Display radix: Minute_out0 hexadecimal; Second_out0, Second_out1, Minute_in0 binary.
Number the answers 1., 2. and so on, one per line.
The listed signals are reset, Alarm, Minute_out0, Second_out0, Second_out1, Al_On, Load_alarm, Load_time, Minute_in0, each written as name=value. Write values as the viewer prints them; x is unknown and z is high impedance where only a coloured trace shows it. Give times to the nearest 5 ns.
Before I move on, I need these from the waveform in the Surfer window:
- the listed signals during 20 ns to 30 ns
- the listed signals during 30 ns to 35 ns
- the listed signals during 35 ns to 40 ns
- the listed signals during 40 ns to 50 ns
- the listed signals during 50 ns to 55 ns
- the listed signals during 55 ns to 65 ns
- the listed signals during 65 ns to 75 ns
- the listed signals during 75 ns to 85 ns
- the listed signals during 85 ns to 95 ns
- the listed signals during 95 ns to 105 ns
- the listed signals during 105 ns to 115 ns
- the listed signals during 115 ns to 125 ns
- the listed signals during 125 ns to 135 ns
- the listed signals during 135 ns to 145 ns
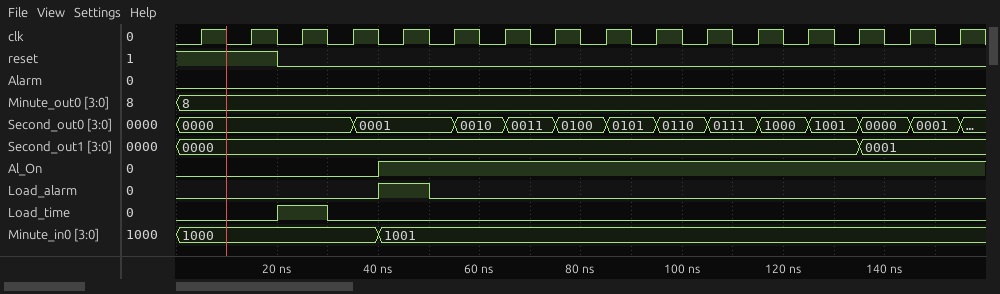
1. reset=0, Alarm=0, Minute_out0=8, Second_out0=0000, Second_out1=0000, Al_On=0, Load_alarm=0, Load_time=1, Minute_in0=1000
2. reset=0, Alarm=0, Minute_out0=8, Second_out0=0000, Second_out1=0000, Al_On=0, Load_alarm=0, Load_time=0, Minute_in0=1000
3. reset=0, Alarm=0, Minute_out0=8, Second_out0=0001, Second_out1=0000, Al_On=0, Load_alarm=0, Load_time=0, Minute_in0=1000
4. reset=0, Alarm=0, Minute_out0=8, Second_out0=0001, Second_out1=0000, Al_On=1, Load_alarm=1, Load_time=0, Minute_in0=1001
5. reset=0, Alarm=0, Minute_out0=8, Second_out0=0001, Second_out1=0000, Al_On=1, Load_alarm=0, Load_time=0, Minute_in0=1001
6. reset=0, Alarm=0, Minute_out0=8, Second_out0=0010, Second_out1=0000, Al_On=1, Load_alarm=0, Load_time=0, Minute_in0=1001
7. reset=0, Alarm=0, Minute_out0=8, Second_out0=0011, Second_out1=0000, Al_On=1, Load_alarm=0, Load_time=0, Minute_in0=1001
8. reset=0, Alarm=0, Minute_out0=8, Second_out0=0100, Second_out1=0000, Al_On=1, Load_alarm=0, Load_time=0, Minute_in0=1001
9. reset=0, Alarm=0, Minute_out0=8, Second_out0=0101, Second_out1=0000, Al_On=1, Load_alarm=0, Load_time=0, Minute_in0=1001
10. reset=0, Alarm=0, Minute_out0=8, Second_out0=0110, Second_out1=0000, Al_On=1, Load_alarm=0, Load_time=0, Minute_in0=1001
11. reset=0, Alarm=0, Minute_out0=8, Second_out0=0111, Second_out1=0000, Al_On=1, Load_alarm=0, Load_time=0, Minute_in0=1001
12. reset=0, Alarm=0, Minute_out0=8, Second_out0=1000, Second_out1=0000, Al_On=1, Load_alarm=0, Load_time=0, Minute_in0=1001
13. reset=0, Alarm=0, Minute_out0=8, Second_out0=1001, Second_out1=0000, Al_On=1, Load_alarm=0, Load_time=0, Minute_in0=1001
14. reset=0, Alarm=0, Minute_out0=8, Second_out0=0000, Second_out1=0001, Al_On=1, Load_alarm=0, Load_time=0, Minute_in0=1001
